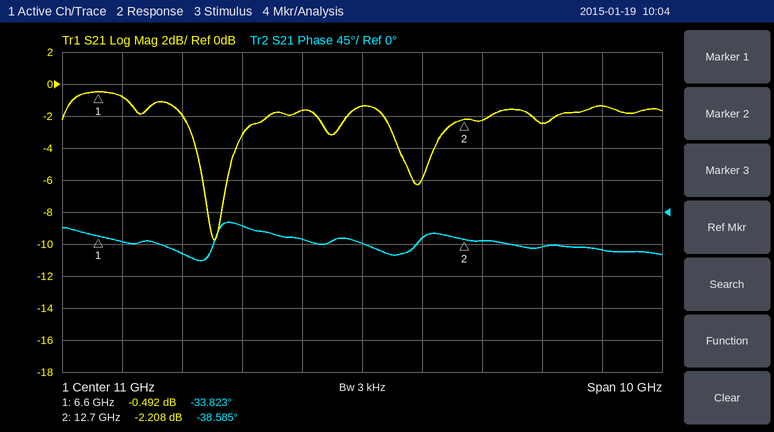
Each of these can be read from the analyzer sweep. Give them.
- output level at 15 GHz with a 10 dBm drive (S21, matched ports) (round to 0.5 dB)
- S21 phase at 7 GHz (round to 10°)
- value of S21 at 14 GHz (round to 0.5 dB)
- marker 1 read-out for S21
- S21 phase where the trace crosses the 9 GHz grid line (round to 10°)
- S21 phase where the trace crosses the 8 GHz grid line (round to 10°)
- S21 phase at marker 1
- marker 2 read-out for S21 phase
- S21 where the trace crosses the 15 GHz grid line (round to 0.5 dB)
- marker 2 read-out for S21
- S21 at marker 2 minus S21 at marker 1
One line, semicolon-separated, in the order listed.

8.5 dBm; -40°; -2.5 dB; -0.492 dB; -20°; -60°; -33.823°; -38.585°; -1.5 dB; -2.208 dB; -1.716 dB
